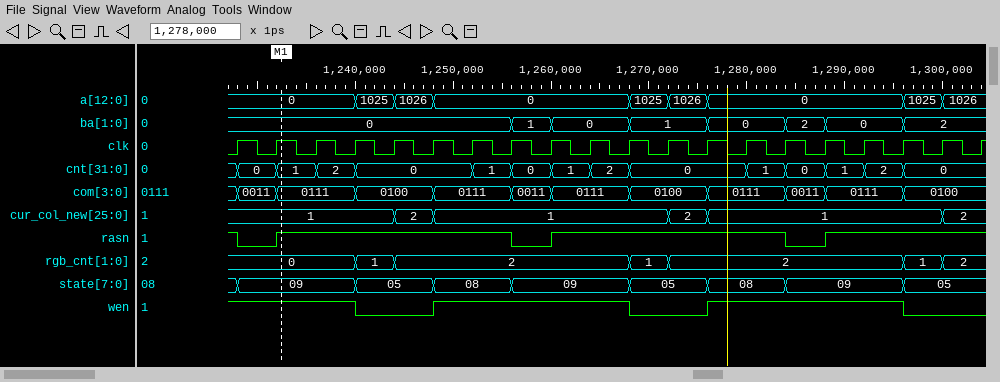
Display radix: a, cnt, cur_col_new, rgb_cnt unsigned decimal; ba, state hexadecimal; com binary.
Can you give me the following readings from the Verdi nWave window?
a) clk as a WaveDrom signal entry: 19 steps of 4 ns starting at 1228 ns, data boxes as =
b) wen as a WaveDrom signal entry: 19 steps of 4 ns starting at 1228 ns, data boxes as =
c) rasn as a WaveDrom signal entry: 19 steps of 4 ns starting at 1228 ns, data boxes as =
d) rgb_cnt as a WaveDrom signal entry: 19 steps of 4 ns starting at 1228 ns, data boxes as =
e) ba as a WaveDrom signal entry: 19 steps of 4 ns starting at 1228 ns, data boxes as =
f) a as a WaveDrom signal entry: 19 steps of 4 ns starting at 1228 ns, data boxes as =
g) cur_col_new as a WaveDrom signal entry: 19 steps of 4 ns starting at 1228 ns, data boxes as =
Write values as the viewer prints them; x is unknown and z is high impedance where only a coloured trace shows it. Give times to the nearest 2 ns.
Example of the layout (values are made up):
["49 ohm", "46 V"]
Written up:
["{name: 'clk', wave: 'p..................'}", "{name: 'wen', wave: '1..0.1....0.1....0.'}", "{name: 'rasn', wave: '01.....01.....01...'}", "{name: 'rgb_cnt', wave: '=..==.....==.....==', data: '0 1 2 1 2 1 2'}", "{name: 'ba', wave: '=......==.=.=.==.=.', data: '0 1 0 1 0 2 0 2'}", "{name: 'a', wave: '=..===....===....==', data: '0 1025 1026 0 1025 1026 0 1025 1026'}", "{name: 'cur_col_new', wave: '=...==.....==.....=', data: '1 2 1 2 1 2'}"]
